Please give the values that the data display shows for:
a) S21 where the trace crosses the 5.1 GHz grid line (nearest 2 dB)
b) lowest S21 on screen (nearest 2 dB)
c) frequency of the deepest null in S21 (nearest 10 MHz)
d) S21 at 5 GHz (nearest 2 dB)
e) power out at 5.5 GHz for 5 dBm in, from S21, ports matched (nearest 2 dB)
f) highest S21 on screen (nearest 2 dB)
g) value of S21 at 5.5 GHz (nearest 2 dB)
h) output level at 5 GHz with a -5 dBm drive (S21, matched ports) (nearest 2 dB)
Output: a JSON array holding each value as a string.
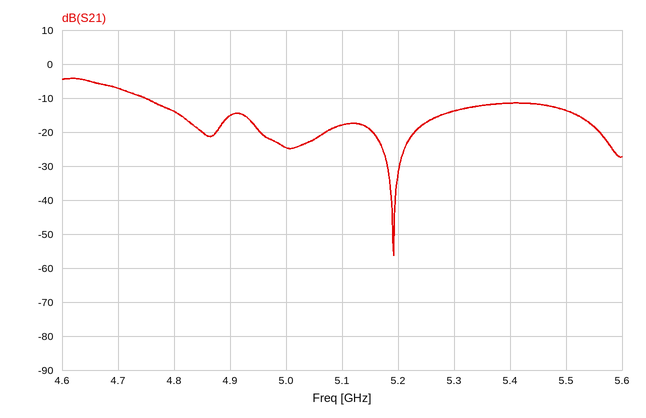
["-18 dB", "-56 dB", "5.19 GHz", "-24 dB", "-8 dBm", "-4 dB", "-14 dB", "-30 dBm"]
